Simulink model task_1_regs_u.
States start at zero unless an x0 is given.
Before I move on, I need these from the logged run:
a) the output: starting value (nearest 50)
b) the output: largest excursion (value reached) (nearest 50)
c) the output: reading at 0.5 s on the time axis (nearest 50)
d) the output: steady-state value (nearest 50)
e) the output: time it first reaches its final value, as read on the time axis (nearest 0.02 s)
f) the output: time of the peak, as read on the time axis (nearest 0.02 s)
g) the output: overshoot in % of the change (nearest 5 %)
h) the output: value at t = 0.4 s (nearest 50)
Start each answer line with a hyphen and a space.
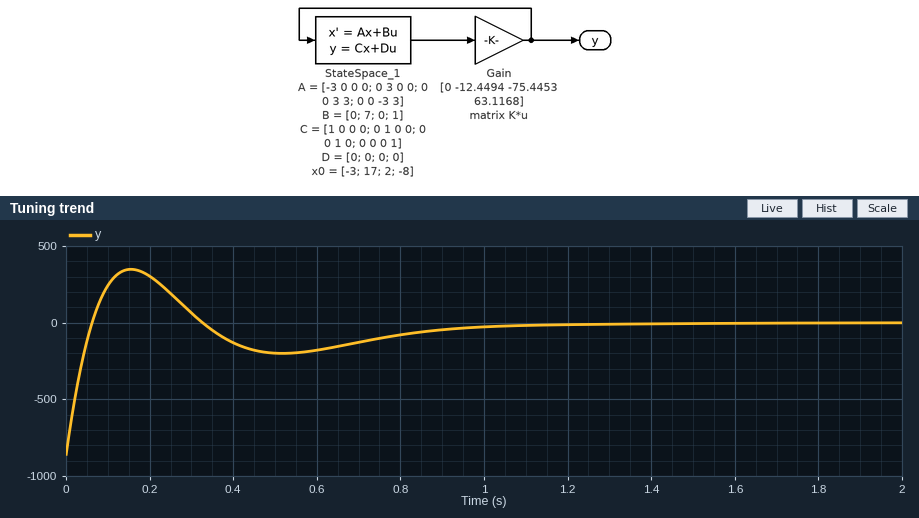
- -850
- 350
- -200
- 0
- 0.06 s
- 0.16 s
- 40 %
- -150
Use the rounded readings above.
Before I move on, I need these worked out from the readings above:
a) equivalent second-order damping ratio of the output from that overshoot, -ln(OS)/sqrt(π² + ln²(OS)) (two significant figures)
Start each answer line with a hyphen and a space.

- 0.28
